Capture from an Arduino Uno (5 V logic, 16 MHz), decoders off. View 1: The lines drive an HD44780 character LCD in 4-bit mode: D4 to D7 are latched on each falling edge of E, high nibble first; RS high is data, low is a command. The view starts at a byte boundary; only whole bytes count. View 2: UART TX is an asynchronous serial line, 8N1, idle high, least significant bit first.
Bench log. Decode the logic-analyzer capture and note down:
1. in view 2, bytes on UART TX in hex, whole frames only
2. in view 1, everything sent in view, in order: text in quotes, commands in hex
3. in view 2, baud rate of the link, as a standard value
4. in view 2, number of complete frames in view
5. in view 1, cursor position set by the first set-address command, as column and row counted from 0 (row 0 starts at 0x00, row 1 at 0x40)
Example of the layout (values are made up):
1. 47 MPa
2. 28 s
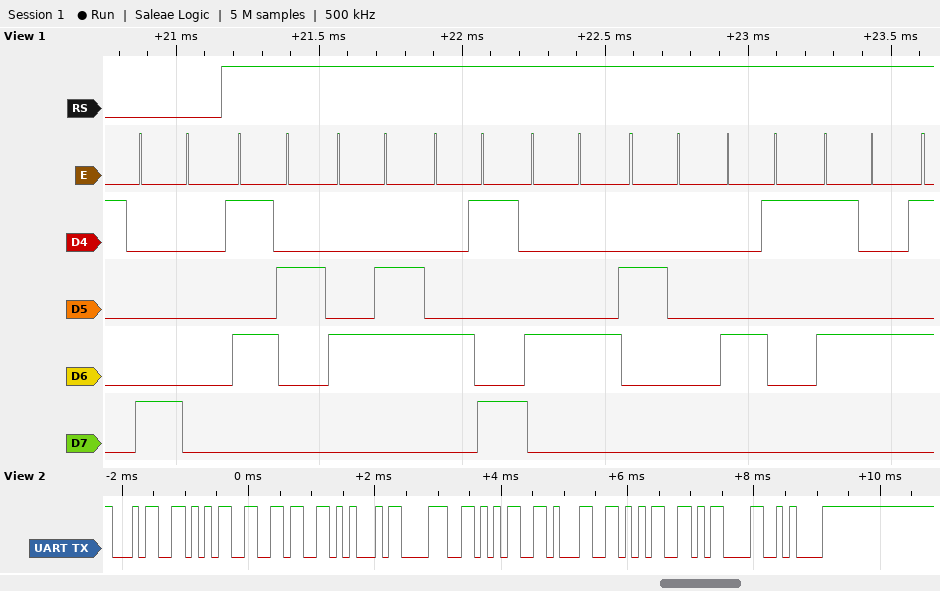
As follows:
1. 0x34 0x35 0x36 0x45 0x38 0x35 0x31 0x35 0x0D 0x0A
2. 0x80 "RFID AT"
3. 9600 baud
4. 10
5. column 0, row 0
